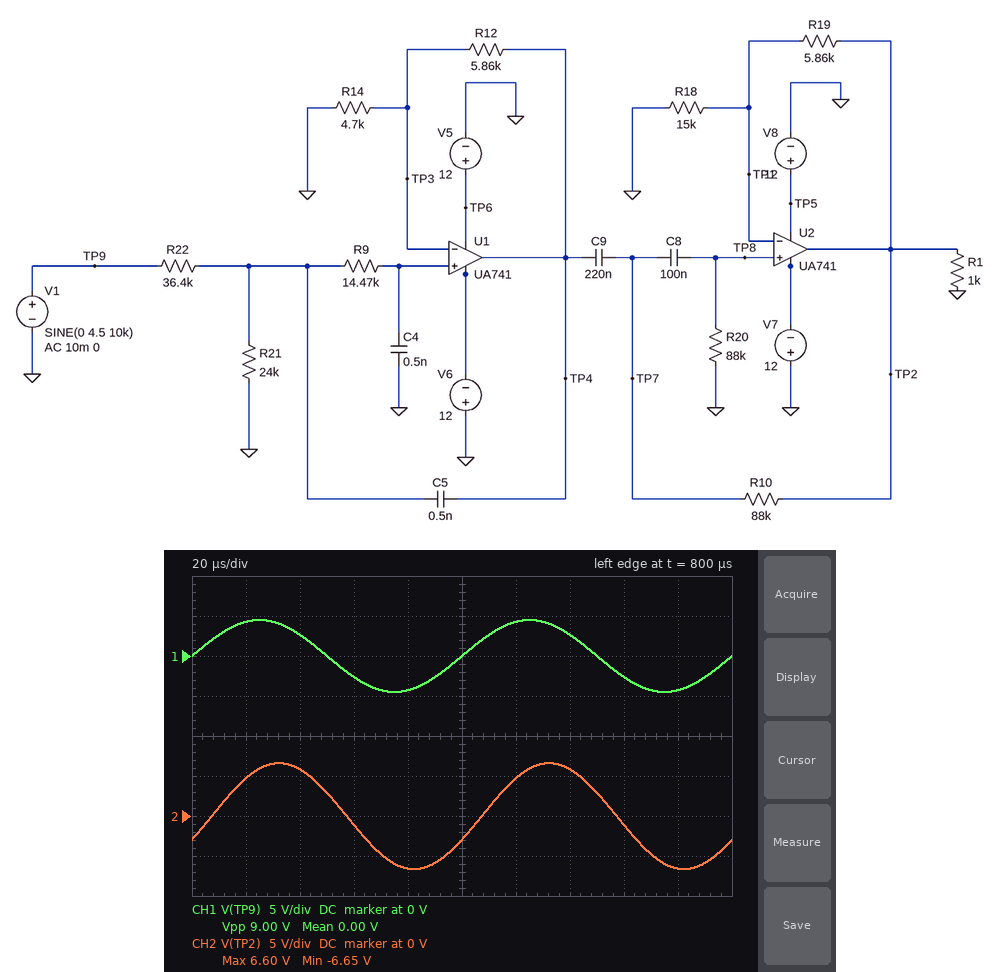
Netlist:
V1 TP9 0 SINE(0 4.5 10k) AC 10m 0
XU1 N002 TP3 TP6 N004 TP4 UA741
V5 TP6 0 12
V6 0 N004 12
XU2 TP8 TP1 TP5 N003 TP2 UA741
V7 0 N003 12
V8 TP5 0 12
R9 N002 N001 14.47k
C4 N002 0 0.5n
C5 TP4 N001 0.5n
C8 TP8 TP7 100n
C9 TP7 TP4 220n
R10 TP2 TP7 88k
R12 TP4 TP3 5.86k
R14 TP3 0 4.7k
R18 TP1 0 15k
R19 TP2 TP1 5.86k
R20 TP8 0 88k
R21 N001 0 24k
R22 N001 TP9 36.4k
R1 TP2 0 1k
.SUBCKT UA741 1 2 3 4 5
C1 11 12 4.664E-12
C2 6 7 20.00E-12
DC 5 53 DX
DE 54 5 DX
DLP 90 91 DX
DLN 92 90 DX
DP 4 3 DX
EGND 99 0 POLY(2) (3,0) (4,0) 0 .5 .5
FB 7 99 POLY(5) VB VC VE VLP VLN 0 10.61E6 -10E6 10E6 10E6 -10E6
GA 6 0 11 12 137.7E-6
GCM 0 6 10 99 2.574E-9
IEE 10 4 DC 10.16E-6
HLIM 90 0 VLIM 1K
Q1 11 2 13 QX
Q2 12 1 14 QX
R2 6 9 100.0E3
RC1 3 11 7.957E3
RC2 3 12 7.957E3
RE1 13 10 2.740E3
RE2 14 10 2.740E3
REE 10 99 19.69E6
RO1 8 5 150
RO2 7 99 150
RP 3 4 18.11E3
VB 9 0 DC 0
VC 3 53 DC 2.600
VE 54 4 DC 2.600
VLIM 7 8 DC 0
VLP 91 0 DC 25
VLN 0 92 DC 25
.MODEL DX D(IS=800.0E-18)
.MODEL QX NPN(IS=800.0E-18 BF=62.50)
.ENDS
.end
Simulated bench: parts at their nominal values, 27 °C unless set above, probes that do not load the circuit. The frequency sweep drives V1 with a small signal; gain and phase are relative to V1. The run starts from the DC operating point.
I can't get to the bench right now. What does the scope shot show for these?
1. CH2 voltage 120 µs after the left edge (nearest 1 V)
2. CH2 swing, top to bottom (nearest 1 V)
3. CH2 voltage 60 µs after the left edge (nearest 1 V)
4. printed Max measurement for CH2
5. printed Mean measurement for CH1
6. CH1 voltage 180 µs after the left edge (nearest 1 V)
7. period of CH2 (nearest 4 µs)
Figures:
5 V
13 V
-1 V
6.60 V
0.00 V
-4 V
100 µs
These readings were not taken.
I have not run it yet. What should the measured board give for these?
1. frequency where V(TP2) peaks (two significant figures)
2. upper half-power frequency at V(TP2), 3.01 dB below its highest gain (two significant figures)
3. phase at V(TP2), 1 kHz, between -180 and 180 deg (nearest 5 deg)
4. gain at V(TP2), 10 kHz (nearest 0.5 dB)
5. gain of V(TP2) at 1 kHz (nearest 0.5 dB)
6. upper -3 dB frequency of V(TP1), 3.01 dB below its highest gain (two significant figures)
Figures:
18 kHz
25 kHz
0 deg
3.5 dB
2.0 dB
25 kHz
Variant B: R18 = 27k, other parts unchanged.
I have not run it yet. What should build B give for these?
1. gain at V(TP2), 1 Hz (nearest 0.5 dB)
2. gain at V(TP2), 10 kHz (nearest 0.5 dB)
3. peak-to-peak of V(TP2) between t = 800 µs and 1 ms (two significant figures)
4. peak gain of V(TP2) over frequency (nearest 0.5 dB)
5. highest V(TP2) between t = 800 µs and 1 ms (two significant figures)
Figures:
-43.0 dB
2.0 dB
12 V
4.0 dB
5.8 V
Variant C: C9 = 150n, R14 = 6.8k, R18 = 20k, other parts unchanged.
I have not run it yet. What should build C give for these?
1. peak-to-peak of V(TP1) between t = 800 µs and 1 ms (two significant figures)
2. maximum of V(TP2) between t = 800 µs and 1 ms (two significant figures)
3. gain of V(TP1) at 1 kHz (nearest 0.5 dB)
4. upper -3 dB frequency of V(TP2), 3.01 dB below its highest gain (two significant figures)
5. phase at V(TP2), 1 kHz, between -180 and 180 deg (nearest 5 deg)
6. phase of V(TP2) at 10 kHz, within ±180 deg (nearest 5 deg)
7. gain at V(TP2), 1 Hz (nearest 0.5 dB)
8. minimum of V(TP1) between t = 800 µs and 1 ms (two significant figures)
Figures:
7.1 V
4.6 V
-2.5 dB
24 kHz
0 deg
-35 deg
-47.0 dB
-3.6 V
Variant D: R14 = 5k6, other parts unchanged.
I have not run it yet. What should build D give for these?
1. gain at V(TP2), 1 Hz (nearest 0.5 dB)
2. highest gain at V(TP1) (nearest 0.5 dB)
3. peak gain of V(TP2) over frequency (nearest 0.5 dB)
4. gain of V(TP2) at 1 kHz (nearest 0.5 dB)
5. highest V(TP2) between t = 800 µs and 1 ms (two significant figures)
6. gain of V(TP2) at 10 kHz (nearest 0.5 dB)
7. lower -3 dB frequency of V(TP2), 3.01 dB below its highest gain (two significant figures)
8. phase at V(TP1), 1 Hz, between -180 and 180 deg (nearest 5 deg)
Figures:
-42.5 dB
0 dB
3.0 dB
1.0 dB
5.7 V
2.0 dB
28 Hz
170 deg
